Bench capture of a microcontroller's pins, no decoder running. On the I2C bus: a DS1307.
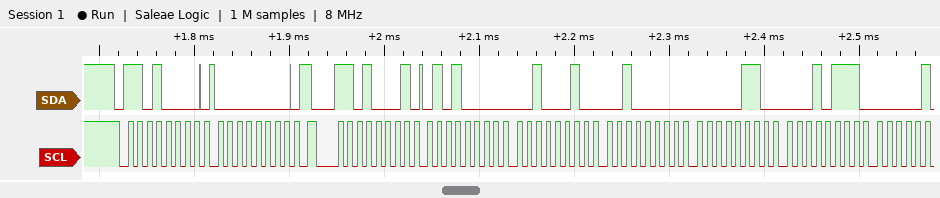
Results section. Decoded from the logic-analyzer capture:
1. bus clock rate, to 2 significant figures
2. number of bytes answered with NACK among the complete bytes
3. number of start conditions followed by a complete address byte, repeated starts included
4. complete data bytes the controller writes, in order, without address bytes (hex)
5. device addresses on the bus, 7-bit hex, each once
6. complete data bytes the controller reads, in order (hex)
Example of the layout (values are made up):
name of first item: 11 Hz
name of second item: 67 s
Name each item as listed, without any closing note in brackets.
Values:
bus clock rate, to 2 significant figures: 100 kHz
number of bytes answered with NACK among the complete bytes: 0
number of start conditions followed by a complete address byte, repeated starts included: 2
complete data bytes the controller writes, in order, without address bytes: 00
device addresses on the bus, 7-bit hex, each once: 0x68
complete data bytes the controller reads, in order: 50 22 20 06 17
